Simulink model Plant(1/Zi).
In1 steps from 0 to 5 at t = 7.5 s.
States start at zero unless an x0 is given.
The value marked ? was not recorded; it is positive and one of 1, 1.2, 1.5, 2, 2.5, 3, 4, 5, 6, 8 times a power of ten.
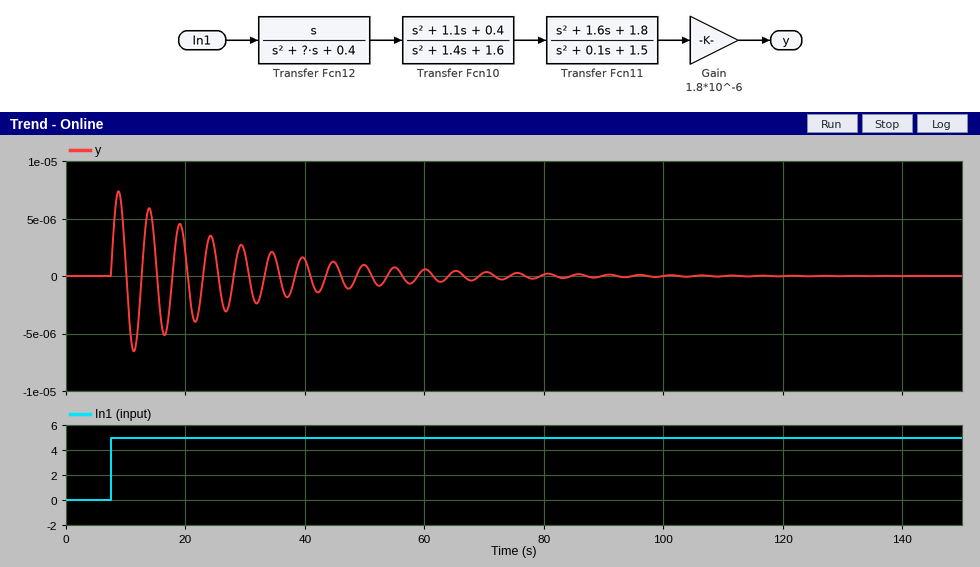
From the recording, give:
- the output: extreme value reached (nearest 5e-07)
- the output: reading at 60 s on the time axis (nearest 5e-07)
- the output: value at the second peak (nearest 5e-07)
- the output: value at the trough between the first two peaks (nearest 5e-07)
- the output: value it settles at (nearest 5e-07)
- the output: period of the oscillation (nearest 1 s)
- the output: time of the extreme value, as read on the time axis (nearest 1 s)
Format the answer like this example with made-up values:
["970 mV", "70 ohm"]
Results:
["0.0000075", "0.0000005", "0.0000060", "-0.0000065", "0.0000000", "5 s", "9 s"]
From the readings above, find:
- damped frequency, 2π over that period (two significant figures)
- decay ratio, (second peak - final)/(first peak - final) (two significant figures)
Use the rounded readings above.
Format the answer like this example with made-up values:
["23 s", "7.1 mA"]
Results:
["1.3 rad/s", "0.80"]
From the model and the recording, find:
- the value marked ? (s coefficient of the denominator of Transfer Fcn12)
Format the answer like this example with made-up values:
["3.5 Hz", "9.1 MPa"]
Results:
["1.2"]
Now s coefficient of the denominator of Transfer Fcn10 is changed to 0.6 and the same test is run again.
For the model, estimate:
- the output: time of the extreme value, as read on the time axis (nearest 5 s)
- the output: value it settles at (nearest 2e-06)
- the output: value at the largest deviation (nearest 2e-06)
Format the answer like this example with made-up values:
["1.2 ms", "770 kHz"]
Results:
["15 s", "0.000000", "0.000014"]
